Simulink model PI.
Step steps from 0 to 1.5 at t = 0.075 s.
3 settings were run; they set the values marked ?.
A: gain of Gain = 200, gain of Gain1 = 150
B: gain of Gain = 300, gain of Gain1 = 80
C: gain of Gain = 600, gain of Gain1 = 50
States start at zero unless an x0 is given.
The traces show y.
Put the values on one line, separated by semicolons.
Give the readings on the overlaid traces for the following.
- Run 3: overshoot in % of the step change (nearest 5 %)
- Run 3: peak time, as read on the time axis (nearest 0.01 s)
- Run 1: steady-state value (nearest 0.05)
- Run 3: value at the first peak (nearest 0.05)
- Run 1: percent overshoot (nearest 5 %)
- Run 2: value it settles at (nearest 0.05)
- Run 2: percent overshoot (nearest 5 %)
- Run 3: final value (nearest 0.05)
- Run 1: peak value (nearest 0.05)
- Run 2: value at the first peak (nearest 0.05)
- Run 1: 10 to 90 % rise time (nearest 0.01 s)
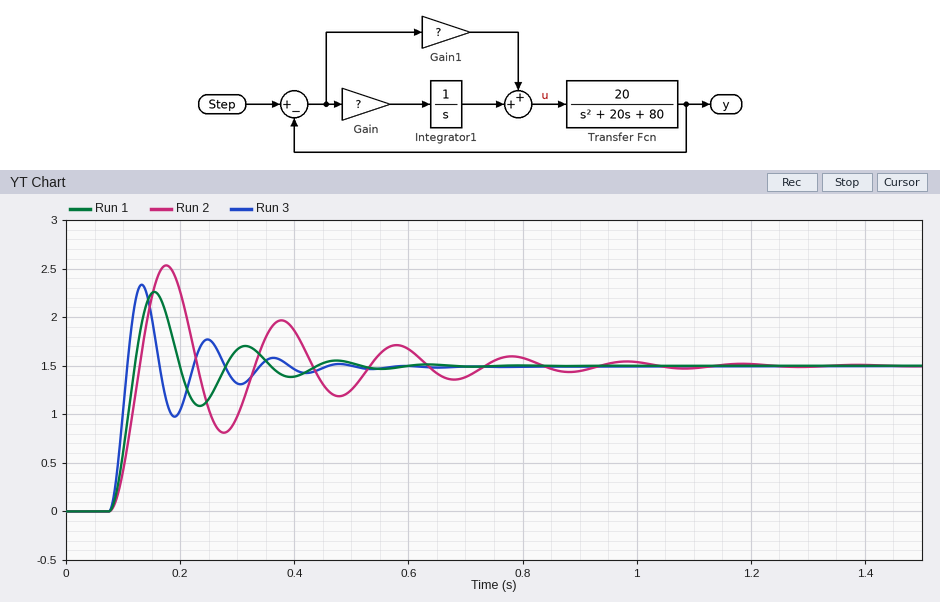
55 %; 0.13 s; 1.50; 2.35; 50 %; 1.50; 70 %; 1.50; 2.25; 2.55; 0.03 s
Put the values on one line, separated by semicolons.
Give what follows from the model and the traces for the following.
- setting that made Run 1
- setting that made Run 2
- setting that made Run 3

B; C; A
